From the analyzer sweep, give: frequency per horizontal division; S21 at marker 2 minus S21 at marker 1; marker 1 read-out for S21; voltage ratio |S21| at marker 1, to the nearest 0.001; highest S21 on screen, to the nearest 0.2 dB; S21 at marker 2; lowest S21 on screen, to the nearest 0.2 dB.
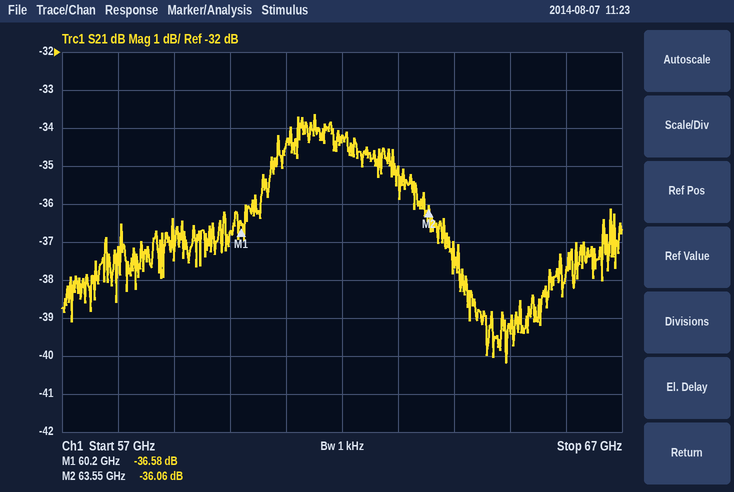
1 GHz
0.52 dB
-36.58 dB
0.015
-33.6 dB
-36.06 dB
-40.2 dB
